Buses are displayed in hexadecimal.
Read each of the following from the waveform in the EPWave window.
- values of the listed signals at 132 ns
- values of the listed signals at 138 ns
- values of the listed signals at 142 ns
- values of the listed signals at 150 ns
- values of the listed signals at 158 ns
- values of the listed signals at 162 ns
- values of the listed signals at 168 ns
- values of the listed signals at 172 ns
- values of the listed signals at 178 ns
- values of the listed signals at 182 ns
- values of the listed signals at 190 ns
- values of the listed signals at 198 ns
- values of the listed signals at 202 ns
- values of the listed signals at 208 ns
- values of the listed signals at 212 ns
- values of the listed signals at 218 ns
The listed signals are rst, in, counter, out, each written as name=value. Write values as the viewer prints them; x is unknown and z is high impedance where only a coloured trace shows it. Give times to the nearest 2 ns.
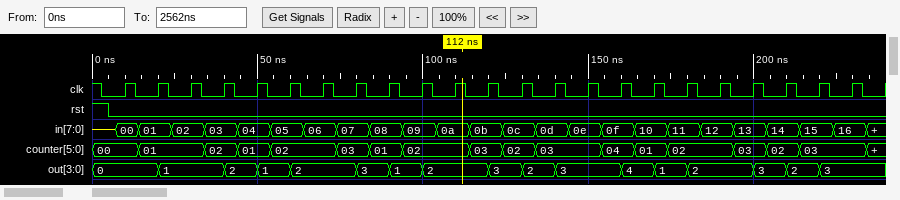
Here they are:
rst=0, in=0c, counter=02, out=2
rst=0, in=0d, counter=03, out=2
rst=0, in=0d, counter=03, out=3
rst=0, in=0e, counter=03, out=3
rst=0, in=0f, counter=04, out=3
rst=0, in=0f, counter=04, out=4
rst=0, in=10, counter=01, out=4
rst=0, in=10, counter=01, out=1
rst=0, in=11, counter=02, out=1
rst=0, in=11, counter=02, out=2
rst=0, in=12, counter=02, out=2
rst=0, in=13, counter=03, out=2
rst=0, in=13, counter=03, out=3
rst=0, in=14, counter=02, out=3
rst=0, in=14, counter=02, out=2
rst=0, in=15, counter=03, out=2
